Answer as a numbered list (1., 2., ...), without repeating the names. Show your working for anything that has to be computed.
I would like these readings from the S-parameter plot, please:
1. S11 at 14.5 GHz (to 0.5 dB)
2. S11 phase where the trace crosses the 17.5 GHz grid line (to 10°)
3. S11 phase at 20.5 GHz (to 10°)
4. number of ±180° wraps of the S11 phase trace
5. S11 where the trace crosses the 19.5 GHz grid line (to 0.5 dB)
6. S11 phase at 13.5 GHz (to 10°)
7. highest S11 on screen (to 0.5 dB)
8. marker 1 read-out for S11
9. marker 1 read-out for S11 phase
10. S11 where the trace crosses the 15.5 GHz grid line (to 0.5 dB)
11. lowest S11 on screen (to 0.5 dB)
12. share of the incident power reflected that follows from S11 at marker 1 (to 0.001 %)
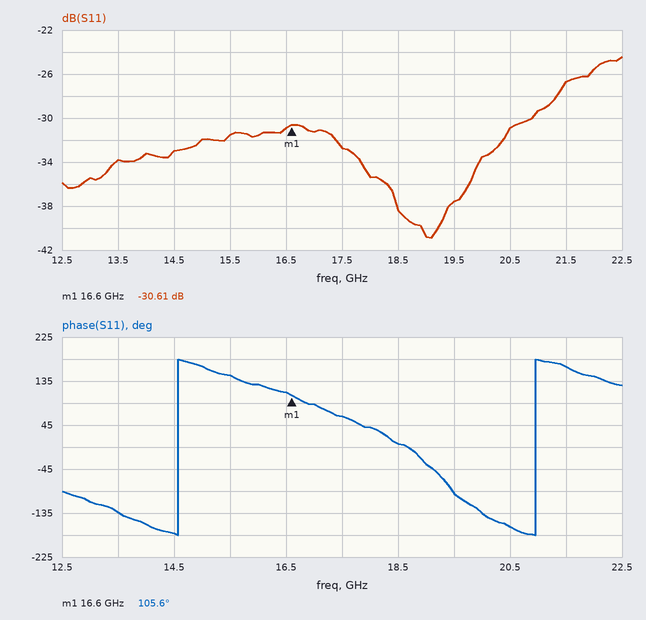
1. -33.0 dB
2. 60°
3. -160°
4. 2
5. -37.5 dB
6. -130°
7. -24.5 dB
8. -30.61 dB
9. 105.6°
10. -31.5 dB
11. -41.0 dB
12. 10^(-30.61/10) ≈ 0.087 %
